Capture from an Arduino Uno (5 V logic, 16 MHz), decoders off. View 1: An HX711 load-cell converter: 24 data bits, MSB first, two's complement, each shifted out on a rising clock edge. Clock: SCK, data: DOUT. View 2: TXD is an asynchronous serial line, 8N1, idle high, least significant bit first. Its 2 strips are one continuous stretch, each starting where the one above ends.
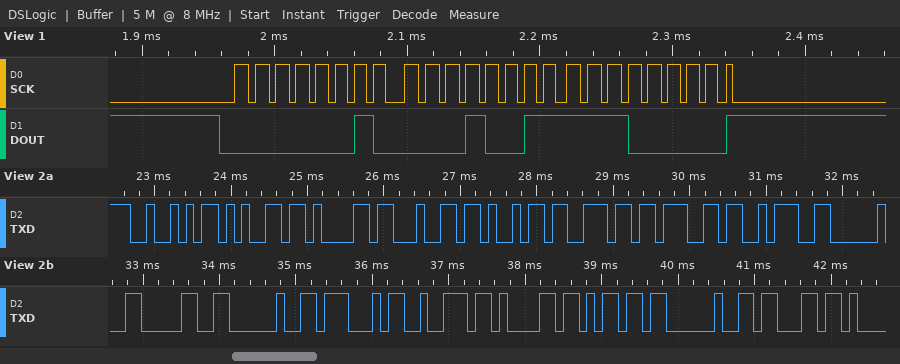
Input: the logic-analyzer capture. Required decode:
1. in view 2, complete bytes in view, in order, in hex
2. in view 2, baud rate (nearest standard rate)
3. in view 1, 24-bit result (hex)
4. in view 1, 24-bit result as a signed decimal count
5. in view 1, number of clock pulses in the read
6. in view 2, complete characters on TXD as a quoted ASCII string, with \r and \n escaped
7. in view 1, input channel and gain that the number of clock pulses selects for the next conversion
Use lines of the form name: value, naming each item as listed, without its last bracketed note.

in view 2, complete bytes in view, in order, in hex: 52 65 61 64 69 6E 67 3A 20 30 20 47 72 61 6D 20 63
in view 2, baud rate: 9600 baud
in view 1, 24-bit result: 0x0213E0
in view 1, 24-bit result as a signed decimal count: 136160
in view 1, number of clock pulses in the read: 25
in view 2, complete characters on TXD as a quoted ASCII string, with \r and \n escaped: "Reading: 0 Gram c"
in view 1, input channel and gain that the number of clock pulses selects for the next conversion: channel A, gain 128
